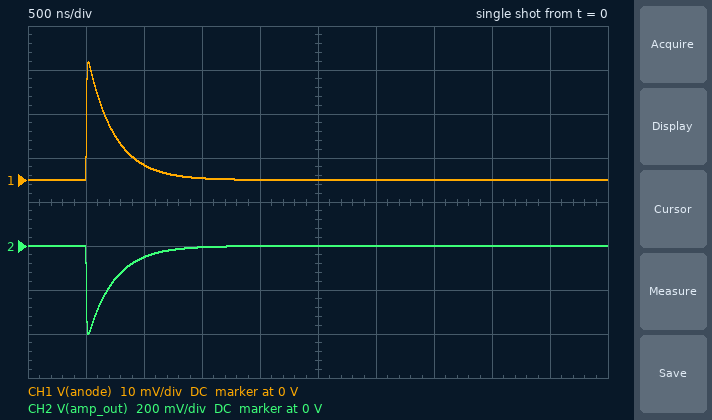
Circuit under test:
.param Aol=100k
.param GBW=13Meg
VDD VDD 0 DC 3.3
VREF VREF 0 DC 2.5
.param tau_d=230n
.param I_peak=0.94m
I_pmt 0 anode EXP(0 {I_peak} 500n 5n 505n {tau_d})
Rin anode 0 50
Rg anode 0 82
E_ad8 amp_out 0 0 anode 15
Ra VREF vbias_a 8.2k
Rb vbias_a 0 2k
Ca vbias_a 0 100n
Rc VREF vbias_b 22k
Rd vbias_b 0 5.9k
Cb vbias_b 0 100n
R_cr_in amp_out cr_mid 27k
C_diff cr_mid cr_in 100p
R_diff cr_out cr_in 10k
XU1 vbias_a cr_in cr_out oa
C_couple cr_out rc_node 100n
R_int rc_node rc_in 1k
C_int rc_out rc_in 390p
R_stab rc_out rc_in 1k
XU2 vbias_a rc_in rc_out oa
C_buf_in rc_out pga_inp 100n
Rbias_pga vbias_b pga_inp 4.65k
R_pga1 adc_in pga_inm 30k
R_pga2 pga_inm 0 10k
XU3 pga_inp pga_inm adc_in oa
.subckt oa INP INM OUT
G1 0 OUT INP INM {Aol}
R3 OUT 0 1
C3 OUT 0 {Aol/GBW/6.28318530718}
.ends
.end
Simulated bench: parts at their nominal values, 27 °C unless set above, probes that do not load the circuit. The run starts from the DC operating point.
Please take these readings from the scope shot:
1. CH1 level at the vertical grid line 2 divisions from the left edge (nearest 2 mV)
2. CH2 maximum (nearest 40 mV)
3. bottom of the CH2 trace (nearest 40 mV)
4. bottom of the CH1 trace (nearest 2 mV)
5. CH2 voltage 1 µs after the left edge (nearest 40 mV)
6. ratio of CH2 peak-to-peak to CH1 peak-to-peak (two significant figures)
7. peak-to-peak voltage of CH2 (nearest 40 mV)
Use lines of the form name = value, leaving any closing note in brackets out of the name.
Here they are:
CH1 level at the vertical grid line 2 divisions from the left edge = 4 mV
CH2 maximum = 0 V
bottom of the CH2 trace = -400 mV
bottom of the CH1 trace = 0 V
CH2 voltage 1 µs after the left edge = -40 mV
ratio of CH2 peak-to-peak to CH1 peak-to-peak = 15
peak-to-peak voltage of CH2 = 400 mV
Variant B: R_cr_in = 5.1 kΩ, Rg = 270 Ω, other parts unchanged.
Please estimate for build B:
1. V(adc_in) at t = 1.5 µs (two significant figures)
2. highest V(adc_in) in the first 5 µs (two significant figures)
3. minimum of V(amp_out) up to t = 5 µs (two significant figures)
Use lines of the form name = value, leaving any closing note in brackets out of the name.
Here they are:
V(adc_in) at t = 1.5 µs = 2.3 V
highest V(adc_in) in the first 5 µs = 2.4 V
minimum of V(amp_out) up to t = 5 µs = -550 mV
